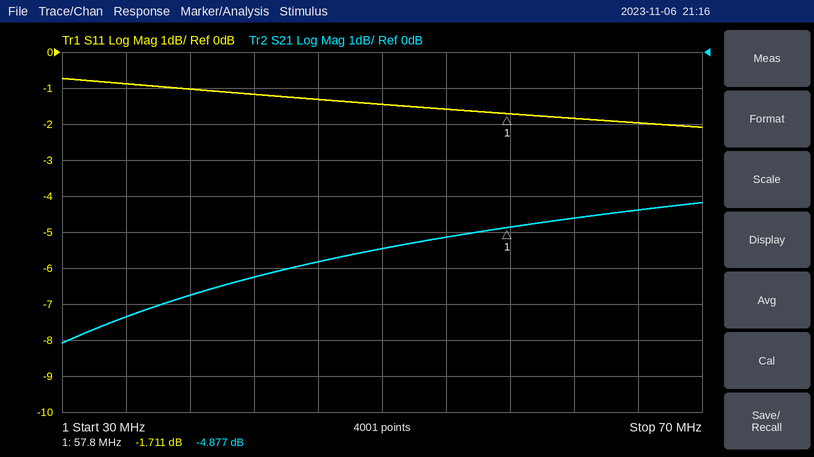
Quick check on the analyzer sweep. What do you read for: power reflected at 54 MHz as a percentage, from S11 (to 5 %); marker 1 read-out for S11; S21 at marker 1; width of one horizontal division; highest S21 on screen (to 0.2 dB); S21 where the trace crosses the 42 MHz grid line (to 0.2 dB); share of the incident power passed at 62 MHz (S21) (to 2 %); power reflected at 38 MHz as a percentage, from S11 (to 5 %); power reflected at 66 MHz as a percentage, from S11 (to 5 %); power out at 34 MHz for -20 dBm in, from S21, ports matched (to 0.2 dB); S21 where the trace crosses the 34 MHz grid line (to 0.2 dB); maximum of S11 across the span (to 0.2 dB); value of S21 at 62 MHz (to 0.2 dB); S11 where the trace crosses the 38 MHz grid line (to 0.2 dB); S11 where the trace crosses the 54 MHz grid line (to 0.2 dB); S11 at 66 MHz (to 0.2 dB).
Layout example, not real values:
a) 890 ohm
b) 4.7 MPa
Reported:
a) 70 %
b) -1.711 dB
c) -4.877 dB
d) 4 MHz
e) -4.2 dB
f) -6.2 dB
g) 34 %
h) 80 %
i) 65 %
j) -27.4 dBm
k) -7.4 dB
l) -0.8 dB
m) -4.6 dB
n) -1.0 dB
o) -1.6 dB
p) -2.0 dB
